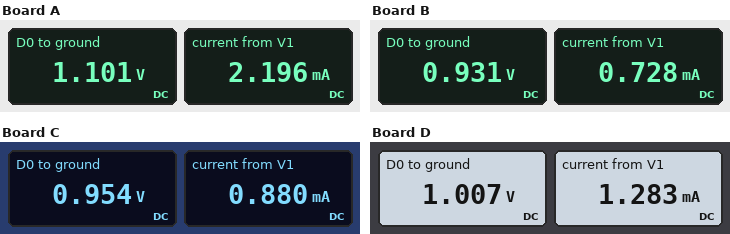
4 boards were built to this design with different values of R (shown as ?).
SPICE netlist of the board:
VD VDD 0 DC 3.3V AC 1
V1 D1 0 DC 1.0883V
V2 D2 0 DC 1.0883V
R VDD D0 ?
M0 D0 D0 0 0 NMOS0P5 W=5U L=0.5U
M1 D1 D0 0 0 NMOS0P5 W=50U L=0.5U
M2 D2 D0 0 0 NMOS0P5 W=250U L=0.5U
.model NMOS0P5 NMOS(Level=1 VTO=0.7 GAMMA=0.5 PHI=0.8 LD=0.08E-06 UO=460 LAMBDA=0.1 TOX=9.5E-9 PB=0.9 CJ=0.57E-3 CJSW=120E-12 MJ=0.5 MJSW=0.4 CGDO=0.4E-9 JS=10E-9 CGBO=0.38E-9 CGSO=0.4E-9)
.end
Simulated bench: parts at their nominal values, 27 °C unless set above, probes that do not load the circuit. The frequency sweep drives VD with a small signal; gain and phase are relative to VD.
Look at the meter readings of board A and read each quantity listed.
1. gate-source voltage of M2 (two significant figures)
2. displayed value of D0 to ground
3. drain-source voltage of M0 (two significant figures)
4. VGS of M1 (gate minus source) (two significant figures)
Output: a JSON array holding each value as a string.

["1.1 V", "1.101 V", "1.1 V", "1.1 V"]
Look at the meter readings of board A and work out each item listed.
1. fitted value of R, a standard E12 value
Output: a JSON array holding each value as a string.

["10 kΩ"]
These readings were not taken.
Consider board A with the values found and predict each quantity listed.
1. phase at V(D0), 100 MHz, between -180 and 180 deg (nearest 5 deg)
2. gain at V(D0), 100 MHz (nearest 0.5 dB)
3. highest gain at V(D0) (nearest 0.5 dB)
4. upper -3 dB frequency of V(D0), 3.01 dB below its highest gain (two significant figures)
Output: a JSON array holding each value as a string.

["-15 deg", "-22.0 dB", "-21.5 dB", "390 MHz"]
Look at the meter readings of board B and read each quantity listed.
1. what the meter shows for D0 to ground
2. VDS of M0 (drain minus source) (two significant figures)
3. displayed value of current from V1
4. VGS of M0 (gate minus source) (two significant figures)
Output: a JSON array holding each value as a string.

["0.931 V", "930 mV", "0.728 mA", "930 mV"]
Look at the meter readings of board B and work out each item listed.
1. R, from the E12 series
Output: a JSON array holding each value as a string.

["33 kΩ"]
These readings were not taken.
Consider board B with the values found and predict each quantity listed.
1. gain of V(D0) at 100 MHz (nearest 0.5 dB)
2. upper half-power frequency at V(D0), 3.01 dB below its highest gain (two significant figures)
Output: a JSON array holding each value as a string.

["-27.5 dB", "210 MHz"]
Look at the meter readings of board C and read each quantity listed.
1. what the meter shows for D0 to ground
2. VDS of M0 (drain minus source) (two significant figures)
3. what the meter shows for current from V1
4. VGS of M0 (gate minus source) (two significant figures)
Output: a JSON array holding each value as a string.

["0.954 V", "950 mV", "0.880 mA", "950 mV"]
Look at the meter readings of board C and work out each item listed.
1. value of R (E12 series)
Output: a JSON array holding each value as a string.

["27 kΩ"]
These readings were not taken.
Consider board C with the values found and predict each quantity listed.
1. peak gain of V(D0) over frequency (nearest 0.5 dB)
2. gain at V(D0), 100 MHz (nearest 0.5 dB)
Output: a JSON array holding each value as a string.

["-26.0 dB", "-26.5 dB"]
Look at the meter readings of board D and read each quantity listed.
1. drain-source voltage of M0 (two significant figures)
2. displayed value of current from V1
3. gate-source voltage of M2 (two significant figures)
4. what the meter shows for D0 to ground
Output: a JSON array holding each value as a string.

["1.0 V", "1.283 mA", "1.0 V", "1.007 V"]
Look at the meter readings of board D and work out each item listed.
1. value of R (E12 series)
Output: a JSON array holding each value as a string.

["18 kΩ"]
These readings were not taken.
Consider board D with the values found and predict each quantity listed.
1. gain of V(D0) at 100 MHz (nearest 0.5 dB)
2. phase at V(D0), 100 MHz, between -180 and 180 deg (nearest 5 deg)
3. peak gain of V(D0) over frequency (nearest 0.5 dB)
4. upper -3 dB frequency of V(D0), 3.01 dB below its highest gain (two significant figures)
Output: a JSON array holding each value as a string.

["-24.5 dB", "-20 deg", "-24.0 dB", "290 MHz"]
